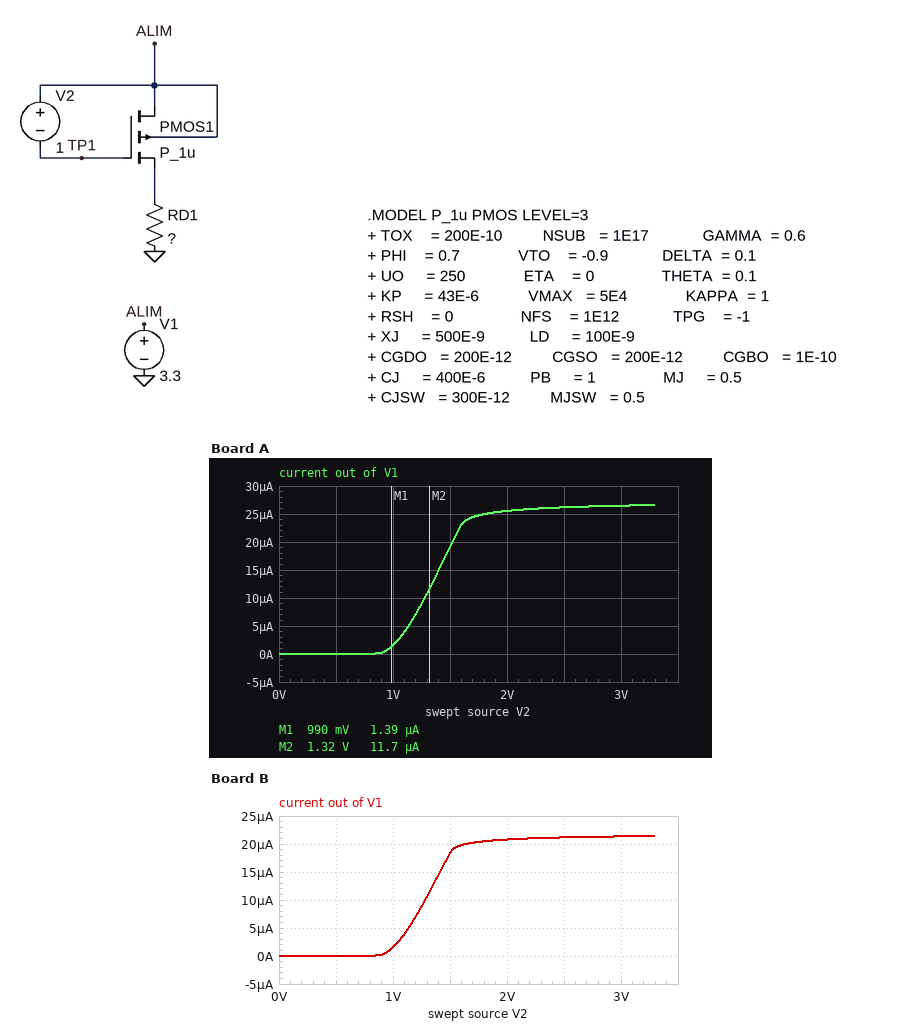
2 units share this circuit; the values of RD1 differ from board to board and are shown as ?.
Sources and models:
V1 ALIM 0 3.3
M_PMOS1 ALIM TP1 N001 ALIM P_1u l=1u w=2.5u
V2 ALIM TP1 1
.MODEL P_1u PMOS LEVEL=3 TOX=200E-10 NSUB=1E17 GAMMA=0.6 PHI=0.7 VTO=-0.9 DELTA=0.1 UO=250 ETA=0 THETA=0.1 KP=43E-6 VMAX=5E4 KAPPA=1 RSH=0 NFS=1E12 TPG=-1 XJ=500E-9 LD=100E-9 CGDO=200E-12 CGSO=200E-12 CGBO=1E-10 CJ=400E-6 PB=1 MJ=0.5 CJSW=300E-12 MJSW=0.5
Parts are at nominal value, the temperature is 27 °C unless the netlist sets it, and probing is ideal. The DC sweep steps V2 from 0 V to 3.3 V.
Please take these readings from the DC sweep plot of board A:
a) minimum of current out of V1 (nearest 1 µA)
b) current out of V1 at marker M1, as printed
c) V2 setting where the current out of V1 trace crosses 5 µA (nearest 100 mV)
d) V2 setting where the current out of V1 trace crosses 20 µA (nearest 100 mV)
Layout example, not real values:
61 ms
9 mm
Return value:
0 A
1.39 µA
1.1 V
1.5 V
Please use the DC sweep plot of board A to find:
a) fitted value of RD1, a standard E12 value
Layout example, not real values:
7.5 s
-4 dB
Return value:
120 kΩ
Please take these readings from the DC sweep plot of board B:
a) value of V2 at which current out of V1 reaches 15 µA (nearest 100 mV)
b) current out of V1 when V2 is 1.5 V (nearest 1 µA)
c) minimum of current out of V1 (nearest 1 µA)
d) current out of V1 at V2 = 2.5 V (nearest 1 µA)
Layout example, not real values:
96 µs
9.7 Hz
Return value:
1.4 V
18 µA
0 A
21 µA
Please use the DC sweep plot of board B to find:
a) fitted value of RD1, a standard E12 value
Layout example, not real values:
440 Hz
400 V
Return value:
150 kΩ
